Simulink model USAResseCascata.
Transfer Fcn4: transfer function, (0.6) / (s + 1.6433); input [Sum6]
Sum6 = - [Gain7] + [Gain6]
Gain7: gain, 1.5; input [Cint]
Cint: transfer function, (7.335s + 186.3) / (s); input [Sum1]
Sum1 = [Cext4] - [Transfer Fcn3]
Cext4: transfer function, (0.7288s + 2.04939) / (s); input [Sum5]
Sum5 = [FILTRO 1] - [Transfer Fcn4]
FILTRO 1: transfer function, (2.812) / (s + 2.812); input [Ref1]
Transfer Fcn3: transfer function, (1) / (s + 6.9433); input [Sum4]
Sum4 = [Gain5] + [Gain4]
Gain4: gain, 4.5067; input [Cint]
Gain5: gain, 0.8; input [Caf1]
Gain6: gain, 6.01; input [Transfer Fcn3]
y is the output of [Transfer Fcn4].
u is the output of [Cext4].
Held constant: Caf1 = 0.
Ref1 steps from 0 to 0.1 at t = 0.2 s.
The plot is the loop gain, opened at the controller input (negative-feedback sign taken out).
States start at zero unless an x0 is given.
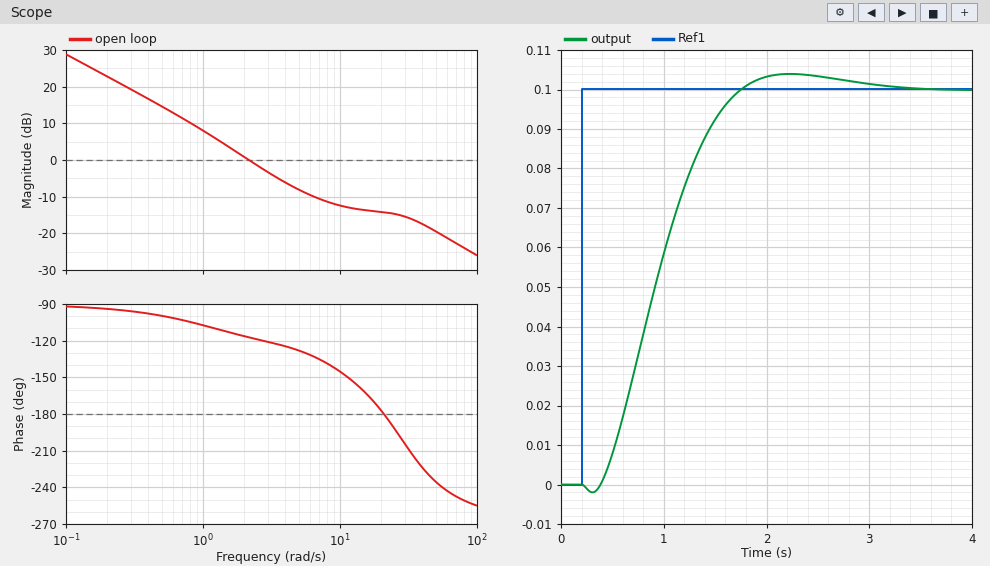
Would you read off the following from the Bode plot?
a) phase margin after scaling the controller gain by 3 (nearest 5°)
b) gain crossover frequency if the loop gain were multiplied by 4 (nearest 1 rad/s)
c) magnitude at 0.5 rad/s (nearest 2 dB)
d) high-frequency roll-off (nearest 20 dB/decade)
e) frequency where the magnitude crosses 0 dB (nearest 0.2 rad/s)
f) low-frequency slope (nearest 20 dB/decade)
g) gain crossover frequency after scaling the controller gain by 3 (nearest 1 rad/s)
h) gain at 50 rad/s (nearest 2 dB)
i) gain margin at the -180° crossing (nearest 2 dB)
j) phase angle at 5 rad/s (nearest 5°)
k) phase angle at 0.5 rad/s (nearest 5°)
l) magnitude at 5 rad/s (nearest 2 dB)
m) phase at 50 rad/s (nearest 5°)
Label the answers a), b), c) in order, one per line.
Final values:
a) 50°
b) 9 rad/s
c) 14 dB
d) -20 dB/decade
e) 2.2 rad/s
f) -20 dB/decade
g) 6 rad/s
h) -20 dB
i) 14 dB
j) -130°
k) -100°
l) -8 dB
m) -235°
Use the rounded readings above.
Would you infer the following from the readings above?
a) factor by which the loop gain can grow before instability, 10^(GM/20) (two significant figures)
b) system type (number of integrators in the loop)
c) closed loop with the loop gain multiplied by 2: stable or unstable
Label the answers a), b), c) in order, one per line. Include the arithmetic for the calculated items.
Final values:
a) 10^(14 / 20) = 5.0
b) 1
c) stable
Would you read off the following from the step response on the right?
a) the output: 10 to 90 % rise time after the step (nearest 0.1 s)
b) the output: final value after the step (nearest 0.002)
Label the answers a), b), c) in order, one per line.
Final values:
a) 0.9 s
b) 0.100
